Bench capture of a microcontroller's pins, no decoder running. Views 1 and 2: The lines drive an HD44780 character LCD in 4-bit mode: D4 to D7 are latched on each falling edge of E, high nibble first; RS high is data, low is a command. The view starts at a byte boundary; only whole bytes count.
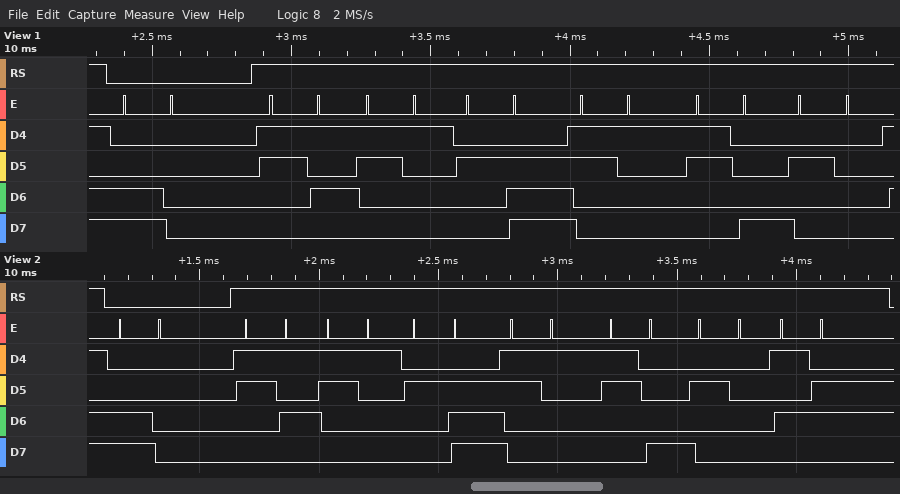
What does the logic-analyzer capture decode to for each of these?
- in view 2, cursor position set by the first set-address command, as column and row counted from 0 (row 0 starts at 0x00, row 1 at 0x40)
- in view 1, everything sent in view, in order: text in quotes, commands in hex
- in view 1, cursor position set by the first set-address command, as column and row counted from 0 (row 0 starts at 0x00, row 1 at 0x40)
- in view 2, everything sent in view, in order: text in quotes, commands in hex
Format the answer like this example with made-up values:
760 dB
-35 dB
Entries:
column 0, row 1
0xC0 "51.18 "
column 0, row 1
0xC0 "51.18 V"
